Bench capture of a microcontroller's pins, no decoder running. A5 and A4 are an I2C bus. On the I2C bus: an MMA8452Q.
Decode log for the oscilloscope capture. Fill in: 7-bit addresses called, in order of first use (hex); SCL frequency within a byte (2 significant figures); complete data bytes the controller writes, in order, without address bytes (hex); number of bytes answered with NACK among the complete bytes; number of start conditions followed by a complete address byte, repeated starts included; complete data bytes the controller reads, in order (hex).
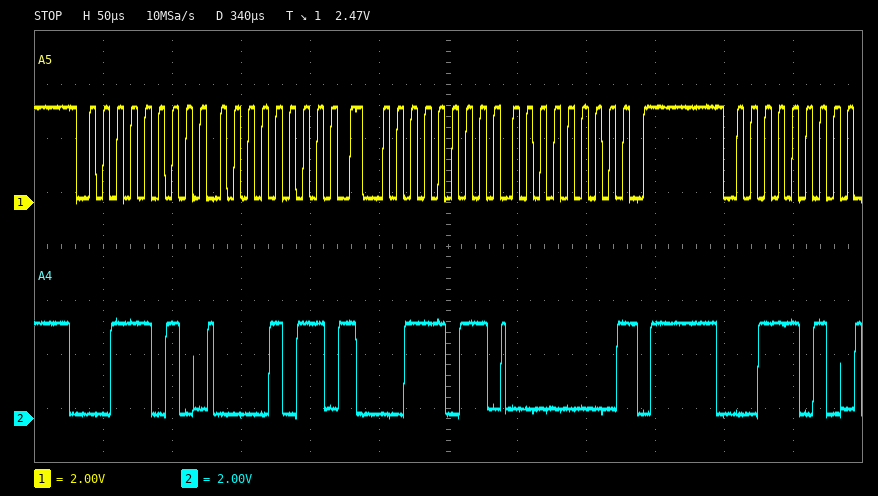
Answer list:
0x1D
100 kHz
0B
1
3
00
